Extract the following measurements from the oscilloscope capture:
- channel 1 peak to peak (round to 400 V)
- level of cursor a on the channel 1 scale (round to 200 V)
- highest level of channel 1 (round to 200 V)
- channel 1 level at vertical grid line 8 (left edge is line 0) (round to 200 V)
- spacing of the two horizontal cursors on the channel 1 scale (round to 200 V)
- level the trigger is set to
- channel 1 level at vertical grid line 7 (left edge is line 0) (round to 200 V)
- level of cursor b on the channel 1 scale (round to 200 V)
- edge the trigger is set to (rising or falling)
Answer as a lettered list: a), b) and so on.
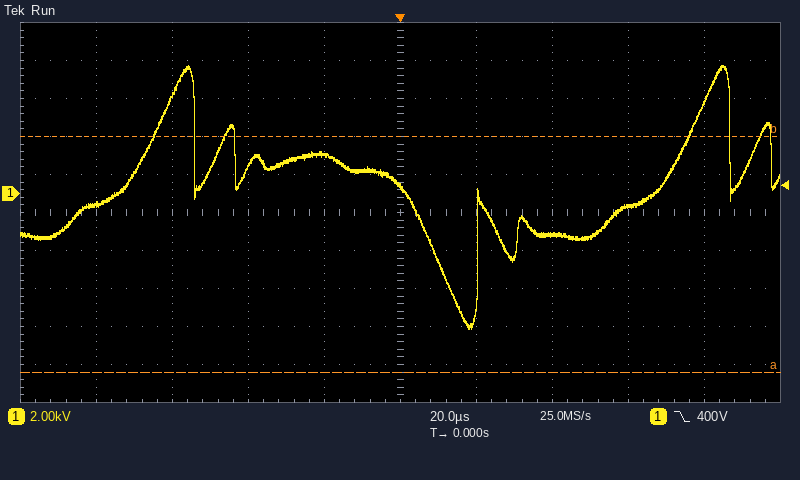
a) 14.0 kV
b) -9.4 kV
c) 6.8 kV
d) -600 V
e) 12.4 kV
f) 400 V
g) -2.2 kV
h) 3.0 kV
i) falling
